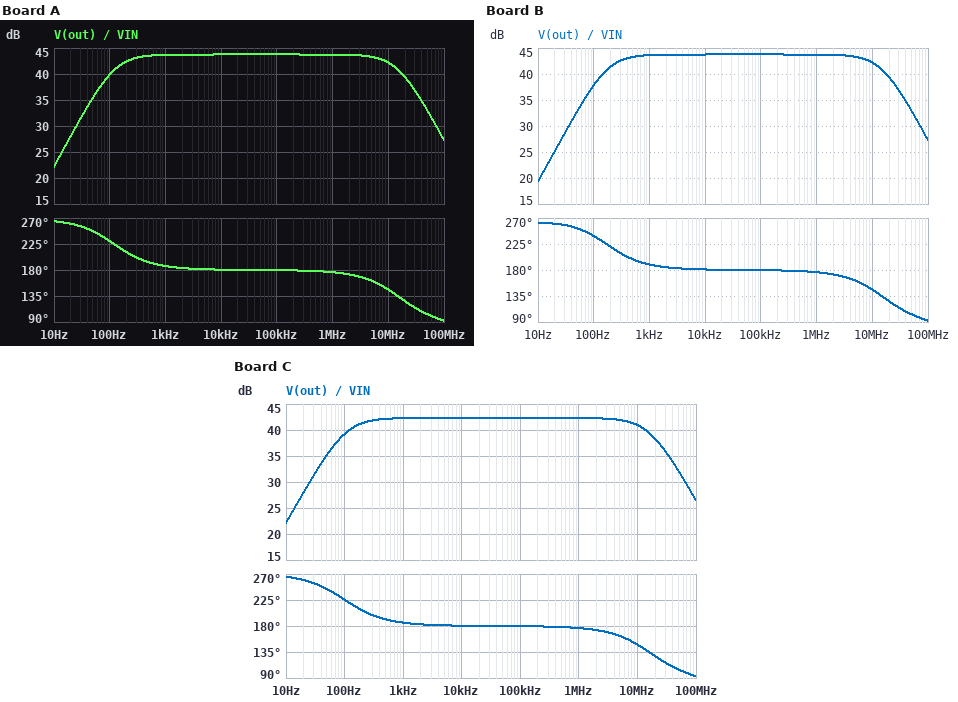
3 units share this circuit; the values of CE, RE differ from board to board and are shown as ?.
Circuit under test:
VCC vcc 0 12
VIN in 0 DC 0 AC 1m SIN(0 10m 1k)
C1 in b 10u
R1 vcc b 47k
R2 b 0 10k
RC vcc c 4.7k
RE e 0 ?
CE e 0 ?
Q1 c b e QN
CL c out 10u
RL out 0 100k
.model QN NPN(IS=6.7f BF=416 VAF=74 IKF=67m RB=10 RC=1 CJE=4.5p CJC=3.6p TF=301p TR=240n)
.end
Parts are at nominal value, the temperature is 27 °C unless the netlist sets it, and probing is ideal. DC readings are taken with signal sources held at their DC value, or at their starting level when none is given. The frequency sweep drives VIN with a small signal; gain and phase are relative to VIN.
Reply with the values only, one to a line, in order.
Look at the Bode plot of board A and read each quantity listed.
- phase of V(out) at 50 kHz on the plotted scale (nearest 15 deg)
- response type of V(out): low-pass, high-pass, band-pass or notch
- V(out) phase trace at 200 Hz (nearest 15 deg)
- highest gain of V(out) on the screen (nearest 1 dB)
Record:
180 deg
band-pass
210 deg
44 dB
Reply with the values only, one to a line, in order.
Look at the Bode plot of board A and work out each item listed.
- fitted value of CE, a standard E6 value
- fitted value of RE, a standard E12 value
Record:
47 µF
1.5 kΩ
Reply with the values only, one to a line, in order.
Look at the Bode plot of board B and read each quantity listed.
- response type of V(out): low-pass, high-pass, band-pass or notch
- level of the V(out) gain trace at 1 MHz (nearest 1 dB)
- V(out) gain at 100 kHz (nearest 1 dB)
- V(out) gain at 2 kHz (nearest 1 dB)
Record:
band-pass
44 dB
44 dB
44 dB
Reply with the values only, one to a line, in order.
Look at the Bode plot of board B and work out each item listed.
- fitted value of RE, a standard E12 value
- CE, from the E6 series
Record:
1.5 kΩ
33 µF
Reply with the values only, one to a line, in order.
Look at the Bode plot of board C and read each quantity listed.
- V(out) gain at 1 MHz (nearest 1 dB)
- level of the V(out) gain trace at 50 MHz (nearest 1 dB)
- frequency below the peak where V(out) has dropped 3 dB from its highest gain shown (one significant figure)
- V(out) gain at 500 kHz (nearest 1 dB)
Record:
42 dB
32 dB
100 Hz
42 dB
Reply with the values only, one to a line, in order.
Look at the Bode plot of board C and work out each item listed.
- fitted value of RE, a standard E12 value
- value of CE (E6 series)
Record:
1.8 kΩ
47 µF
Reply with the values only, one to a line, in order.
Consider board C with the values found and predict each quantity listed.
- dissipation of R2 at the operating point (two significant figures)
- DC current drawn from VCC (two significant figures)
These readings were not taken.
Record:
440 µW
1.0 mA
